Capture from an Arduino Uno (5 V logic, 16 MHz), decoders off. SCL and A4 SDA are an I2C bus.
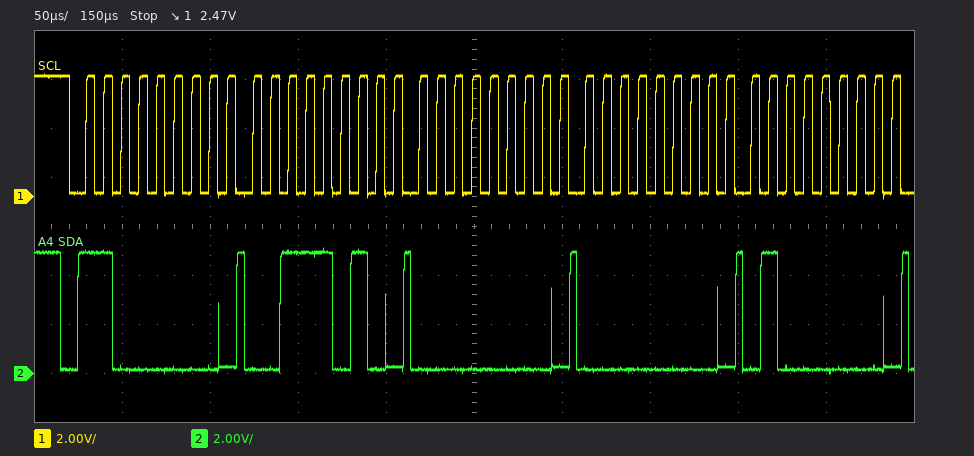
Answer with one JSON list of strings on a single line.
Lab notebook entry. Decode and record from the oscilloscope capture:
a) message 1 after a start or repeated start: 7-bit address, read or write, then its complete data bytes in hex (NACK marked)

["0x60 write: 3A 00 00 40"]
